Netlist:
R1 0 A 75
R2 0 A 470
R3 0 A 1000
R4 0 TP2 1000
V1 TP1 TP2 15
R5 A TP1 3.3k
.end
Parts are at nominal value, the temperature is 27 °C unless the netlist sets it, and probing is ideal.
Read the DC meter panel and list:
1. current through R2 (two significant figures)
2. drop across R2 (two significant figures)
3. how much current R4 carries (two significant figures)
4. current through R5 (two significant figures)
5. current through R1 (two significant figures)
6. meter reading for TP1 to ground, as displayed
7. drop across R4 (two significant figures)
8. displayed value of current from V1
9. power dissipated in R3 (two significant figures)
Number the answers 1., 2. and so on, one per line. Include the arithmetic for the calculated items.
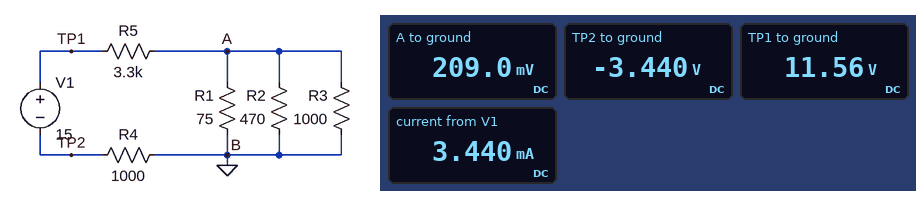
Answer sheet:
1. (209 mV) / 470 Ω = 440 µA
2. 209 mV = 210 mV
3. (0 V - (-3.44 V)) / 1 kΩ = 3.4 mA
4. (11.56 V - 209 mV) / 3.3 kΩ = 3.4 mA
5. (209 mV) / 75 Ω = 2.8 mA
6. 11.56 V
7. 0 V - (-3.44 V) = 3.4 V
8. 3.440 mA
9. (209 mV)^2 / 1 kΩ = 44 µW
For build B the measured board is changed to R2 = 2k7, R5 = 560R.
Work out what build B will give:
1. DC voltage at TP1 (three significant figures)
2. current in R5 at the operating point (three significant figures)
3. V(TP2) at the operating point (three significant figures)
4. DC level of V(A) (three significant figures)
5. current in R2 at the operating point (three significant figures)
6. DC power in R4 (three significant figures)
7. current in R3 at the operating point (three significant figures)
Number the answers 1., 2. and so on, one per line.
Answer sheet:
1. 5.79 V
2. 9.21 mA
3. -9.21 V
4. 627 mV
5. 232 µA
6. 84.9 mW
7. 627 µA
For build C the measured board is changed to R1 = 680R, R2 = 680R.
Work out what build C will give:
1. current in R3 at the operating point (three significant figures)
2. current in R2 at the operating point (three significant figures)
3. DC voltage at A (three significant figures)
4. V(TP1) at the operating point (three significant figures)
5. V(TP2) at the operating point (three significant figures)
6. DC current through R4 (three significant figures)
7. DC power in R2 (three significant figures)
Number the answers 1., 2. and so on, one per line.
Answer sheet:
1. 836 µA
2. 1.23 mA
3. 836 mV
4. 11.7 V
5. -3.29 V
6. 3.29 mA
7. 1.03 mW
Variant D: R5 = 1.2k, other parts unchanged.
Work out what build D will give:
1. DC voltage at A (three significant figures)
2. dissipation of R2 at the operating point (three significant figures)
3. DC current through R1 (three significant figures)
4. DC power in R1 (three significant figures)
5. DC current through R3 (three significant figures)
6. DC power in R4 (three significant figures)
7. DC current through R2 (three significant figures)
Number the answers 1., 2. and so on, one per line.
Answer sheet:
1. 403 mV
2. 346 µW
3. 5.37 mA
4. 2.17 mW
5. 403 µA
6. 44.0 mW
7. 858 µA
